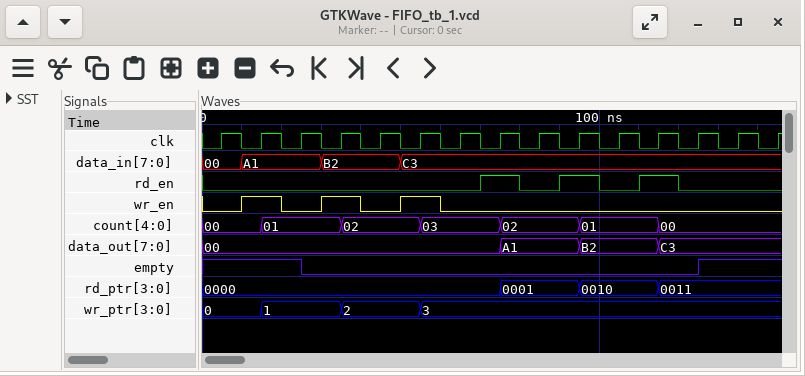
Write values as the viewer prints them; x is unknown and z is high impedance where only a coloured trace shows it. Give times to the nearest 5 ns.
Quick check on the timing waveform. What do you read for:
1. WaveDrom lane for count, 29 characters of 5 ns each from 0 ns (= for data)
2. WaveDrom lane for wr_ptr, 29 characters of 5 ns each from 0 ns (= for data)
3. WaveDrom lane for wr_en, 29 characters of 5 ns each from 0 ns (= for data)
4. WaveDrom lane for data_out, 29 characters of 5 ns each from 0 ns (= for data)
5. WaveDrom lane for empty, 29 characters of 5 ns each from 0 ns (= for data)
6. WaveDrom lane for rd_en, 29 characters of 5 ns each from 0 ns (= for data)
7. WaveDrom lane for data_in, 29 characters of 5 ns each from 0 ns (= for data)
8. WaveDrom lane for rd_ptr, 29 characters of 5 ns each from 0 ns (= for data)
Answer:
{name: 'count', wave: '=..=...=...=...=...=...=.....', data: '00 01 02 03 02 01 00'}
{name: 'wr_ptr', wave: '=..=...=...=.................', data: '0 1 2 3'}
{name: 'wr_en', wave: '0.1.0.1.0.1.0................'}
{name: 'data_out', wave: '=..............=...=...=.....', data: '00 A1 B2 C3'}
{name: 'empty', wave: '1....0...................1...'}
{name: 'rd_en', wave: '0.............1.0.1.0.1.0....'}
{name: 'data_in', wave: '=.=...=...=..................', data: '00 A1 B2 C3'}
{name: 'rd_ptr', wave: '=..............=...=...=.....', data: '0000 0001 0010 0011'}
